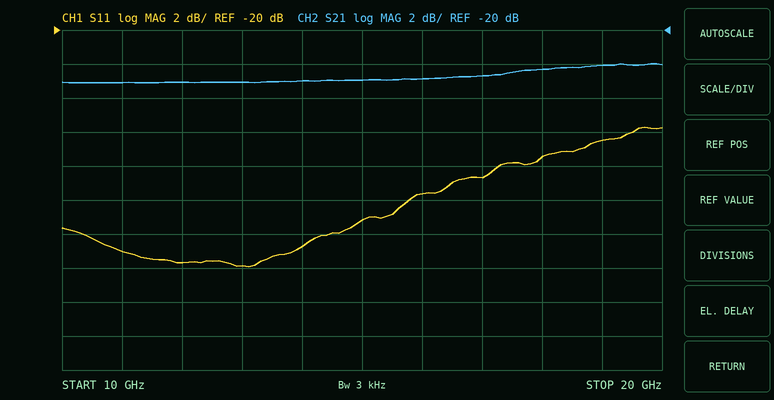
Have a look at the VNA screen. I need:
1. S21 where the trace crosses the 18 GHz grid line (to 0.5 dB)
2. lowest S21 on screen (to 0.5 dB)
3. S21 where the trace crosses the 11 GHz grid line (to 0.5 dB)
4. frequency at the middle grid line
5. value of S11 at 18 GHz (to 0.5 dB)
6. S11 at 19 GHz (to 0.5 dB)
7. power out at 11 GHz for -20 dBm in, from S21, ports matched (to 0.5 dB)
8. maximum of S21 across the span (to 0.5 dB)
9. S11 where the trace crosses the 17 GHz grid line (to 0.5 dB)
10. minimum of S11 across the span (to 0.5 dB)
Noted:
-22.5 dB
-23.0 dB
-23.0 dB
15 GHz
-27.5 dB
-26.5 dB
-43.0 dBm
-22.0 dB
-28.5 dB
-34.0 dB
